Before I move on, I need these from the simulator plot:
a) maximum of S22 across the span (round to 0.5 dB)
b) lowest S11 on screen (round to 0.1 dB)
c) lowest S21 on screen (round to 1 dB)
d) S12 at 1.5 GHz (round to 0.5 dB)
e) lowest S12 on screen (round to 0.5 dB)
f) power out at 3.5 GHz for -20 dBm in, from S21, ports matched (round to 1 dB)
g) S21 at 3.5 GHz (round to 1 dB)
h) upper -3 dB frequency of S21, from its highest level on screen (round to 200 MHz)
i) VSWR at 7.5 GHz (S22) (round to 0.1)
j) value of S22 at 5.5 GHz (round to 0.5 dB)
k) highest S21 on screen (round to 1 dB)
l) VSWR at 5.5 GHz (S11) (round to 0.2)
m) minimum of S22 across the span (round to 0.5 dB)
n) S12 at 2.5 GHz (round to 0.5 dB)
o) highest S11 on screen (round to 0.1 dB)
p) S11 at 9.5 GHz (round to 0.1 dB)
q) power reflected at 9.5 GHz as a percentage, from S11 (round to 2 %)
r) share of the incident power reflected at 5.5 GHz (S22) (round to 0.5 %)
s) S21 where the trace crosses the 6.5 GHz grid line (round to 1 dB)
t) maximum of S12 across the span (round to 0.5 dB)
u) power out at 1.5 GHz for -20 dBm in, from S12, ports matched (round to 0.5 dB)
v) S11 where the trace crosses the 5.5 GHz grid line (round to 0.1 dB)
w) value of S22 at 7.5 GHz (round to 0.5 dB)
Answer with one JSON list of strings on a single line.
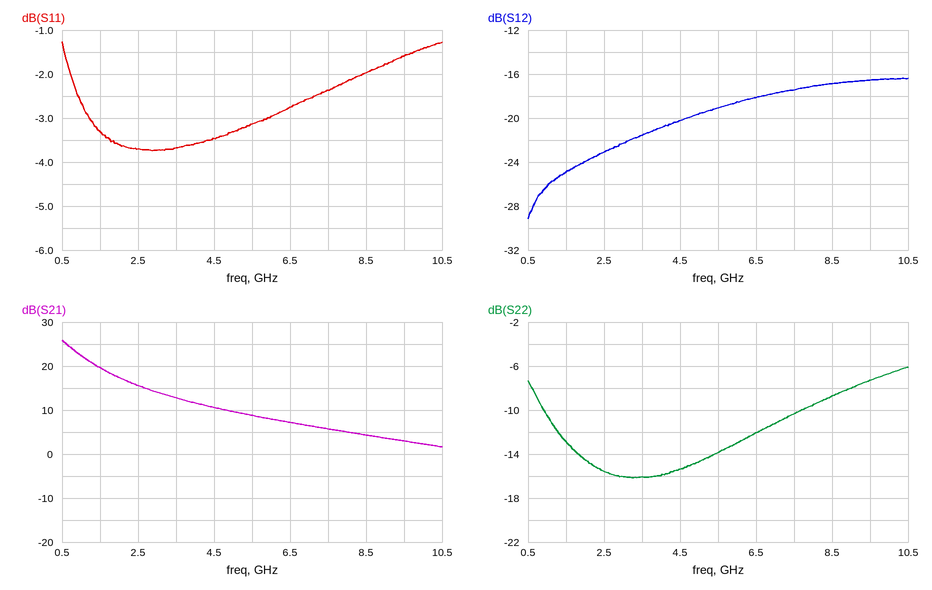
["-6.0 dB", "-3.7 dB", "2 dB", "-25.0 dB", "-29.0 dB", "-7 dBm", "13 dB", "1.0 GHz", "1.9", "-14.0 dB", "26 dB", "5.6", "-16.0 dB", "-23.0 dB", "-1.3 dB", "-1.6 dB", "70 %", "4.0 %", "7 dB", "-16.5 dB", "-45.0 dBm", "-3.1 dB", "-10.5 dB"]
